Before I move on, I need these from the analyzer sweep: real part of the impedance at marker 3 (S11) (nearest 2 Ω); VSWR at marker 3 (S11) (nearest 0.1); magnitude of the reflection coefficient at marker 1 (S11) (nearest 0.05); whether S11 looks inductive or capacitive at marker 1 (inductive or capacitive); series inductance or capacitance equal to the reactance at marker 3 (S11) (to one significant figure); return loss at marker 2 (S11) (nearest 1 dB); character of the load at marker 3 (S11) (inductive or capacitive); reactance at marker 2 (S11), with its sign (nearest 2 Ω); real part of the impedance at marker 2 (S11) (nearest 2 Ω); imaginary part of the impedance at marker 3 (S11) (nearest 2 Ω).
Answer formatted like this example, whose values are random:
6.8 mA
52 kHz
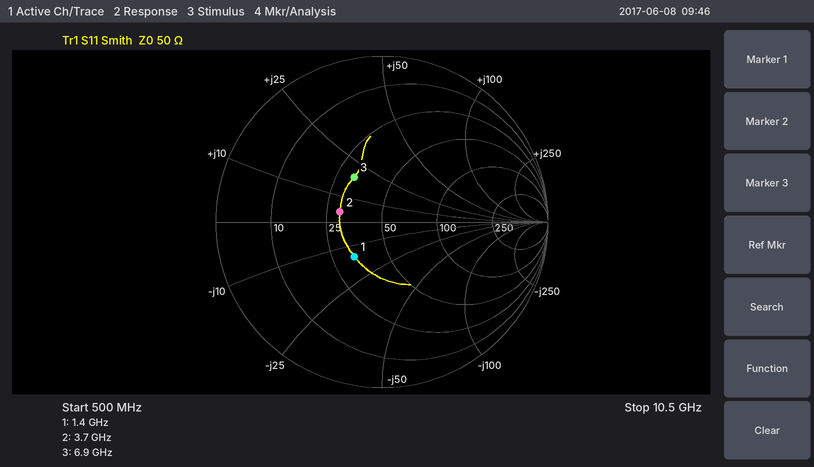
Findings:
32 Ω
1.9
0.25
capacitive
400 pH
12 dB
inductive
+4 Ω
30 Ω
+18 Ω
